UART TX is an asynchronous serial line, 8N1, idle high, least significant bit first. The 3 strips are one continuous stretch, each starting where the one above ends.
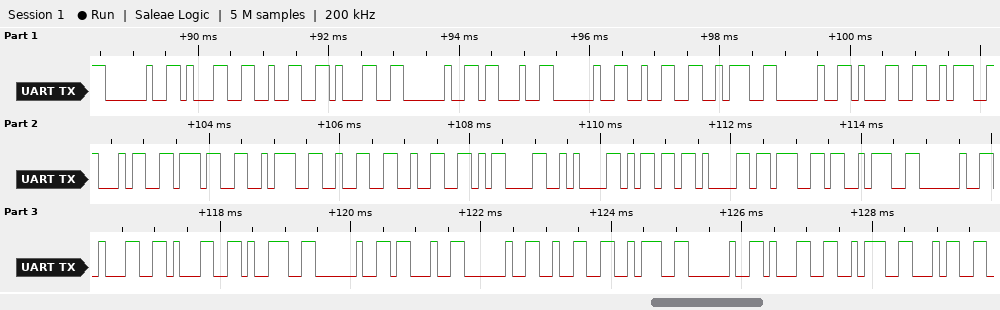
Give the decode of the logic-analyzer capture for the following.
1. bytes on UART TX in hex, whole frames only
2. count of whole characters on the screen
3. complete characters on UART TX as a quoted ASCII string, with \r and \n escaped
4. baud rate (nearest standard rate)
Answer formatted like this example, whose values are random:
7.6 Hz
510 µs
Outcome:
20 31 32 31 20 23 20 32 3A 20 31 3A 34 37 3A 32 32 0D 0A 6D 61 67 3A 20 31 31 39 20 23 20 32 3A 20 31 3A 34
36
" 121 # 2: 1:47:22\r\nmag: 119 # 2: 1:4"
9600 baud
